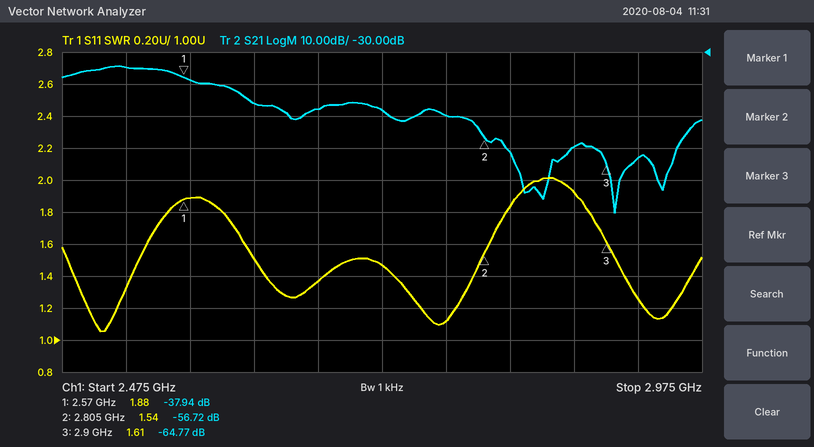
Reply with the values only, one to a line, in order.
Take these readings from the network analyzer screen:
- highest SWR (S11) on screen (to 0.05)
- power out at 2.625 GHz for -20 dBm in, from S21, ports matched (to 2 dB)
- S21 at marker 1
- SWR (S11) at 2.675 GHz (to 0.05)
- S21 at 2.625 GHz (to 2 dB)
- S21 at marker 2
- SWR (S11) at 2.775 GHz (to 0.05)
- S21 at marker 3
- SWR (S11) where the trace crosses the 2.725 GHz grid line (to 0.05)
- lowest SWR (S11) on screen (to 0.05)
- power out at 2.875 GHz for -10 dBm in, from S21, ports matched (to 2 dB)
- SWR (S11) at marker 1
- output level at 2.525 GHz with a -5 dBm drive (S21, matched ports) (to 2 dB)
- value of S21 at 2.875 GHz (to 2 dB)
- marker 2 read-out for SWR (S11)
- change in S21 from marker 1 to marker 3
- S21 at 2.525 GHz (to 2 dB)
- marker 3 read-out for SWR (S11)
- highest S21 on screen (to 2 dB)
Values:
2.00
-66 dBm
-37.94 dB
1.35
-46 dB
-56.72 dB
1.10
-64.77 dB
1.45
1.05
-70 dBm
1.88
-40 dBm
-60 dB
1.54
-26.83 dB
-34 dB
1.61
-34 dB
